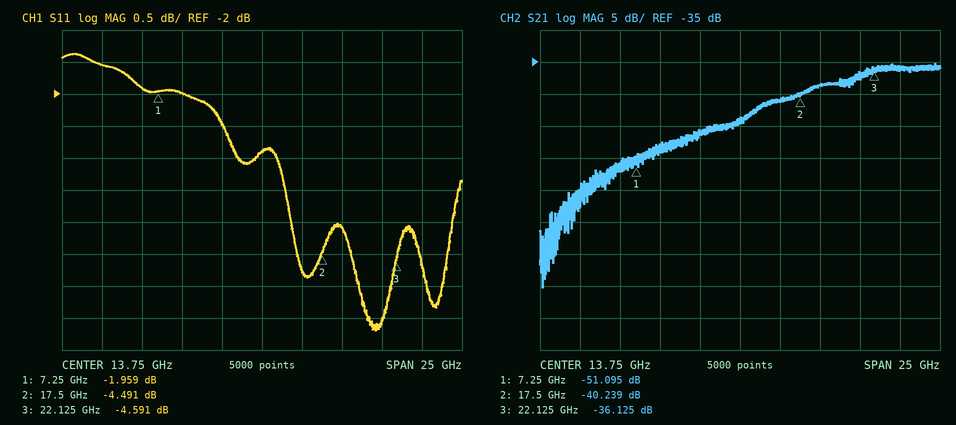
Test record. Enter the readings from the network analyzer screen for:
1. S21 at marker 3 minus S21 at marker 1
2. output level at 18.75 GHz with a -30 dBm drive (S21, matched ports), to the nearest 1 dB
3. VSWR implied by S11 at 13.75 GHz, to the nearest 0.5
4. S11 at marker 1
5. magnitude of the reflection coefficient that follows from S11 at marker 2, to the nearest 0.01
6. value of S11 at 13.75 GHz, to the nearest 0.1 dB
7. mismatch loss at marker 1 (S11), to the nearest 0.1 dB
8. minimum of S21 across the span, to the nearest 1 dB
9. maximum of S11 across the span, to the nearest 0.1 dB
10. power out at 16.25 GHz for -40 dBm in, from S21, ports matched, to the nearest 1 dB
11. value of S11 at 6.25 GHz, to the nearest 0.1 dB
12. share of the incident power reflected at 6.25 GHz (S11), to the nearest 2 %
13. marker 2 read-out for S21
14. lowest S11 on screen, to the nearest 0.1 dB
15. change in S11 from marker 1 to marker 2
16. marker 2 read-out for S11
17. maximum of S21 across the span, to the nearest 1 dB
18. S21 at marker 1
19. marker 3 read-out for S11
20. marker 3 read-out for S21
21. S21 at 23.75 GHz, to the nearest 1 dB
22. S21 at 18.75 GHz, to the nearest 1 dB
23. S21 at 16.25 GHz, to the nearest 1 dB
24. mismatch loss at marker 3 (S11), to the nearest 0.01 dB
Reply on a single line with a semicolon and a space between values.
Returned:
14.970 dB; -69 dBm; 6.0; -1.959 dB; 0.60; -2.9 dB; 4.4 dB; -70 dB; -1.4 dB; -81 dBm; -1.9 dB; 64 %; -40.239 dB; -5.7 dB; -2.532 dB; -4.491 dB; -35 dB; -51.095 dB; -4.591 dB; -36.125 dB; -36 dB; -39 dB; -41 dB; 1.85 dB
